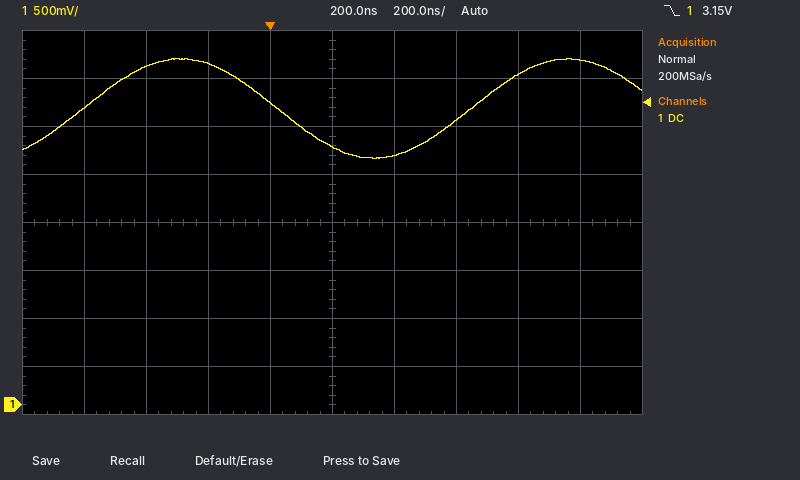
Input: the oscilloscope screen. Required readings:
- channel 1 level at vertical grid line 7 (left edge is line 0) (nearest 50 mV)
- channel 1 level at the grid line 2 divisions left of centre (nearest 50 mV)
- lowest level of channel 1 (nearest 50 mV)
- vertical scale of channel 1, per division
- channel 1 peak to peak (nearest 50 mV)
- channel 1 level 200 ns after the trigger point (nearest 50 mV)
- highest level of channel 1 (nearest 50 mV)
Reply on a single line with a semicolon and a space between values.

2.95 V; 3.55 V; 2.55 V; 500 mV; 1.05 V; 2.70 V; 3.60 V
